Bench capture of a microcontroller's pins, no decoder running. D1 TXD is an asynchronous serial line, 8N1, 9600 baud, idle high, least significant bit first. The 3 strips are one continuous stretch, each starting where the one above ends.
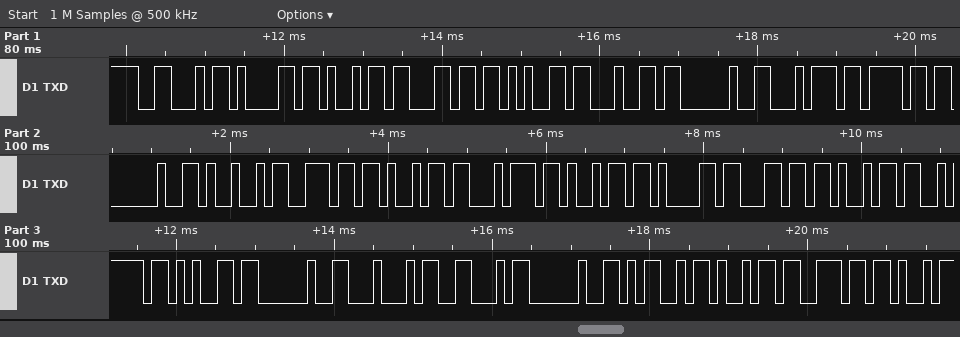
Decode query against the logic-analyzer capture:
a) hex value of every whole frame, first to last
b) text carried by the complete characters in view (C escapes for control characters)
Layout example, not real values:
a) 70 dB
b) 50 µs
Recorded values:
a) 0x46 0x61 0x69 0x6C 0x65 0x64 0x20 0x74 0x6F 0x20 0x49 0x6E 0x69 0x74 0x69 0x61 0x6C 0x69 0x7A 0x65 0x20 0x44 0x46 0x20 0x4D 0x69 0x6E
b) "Failed to Initialize DF Min"
